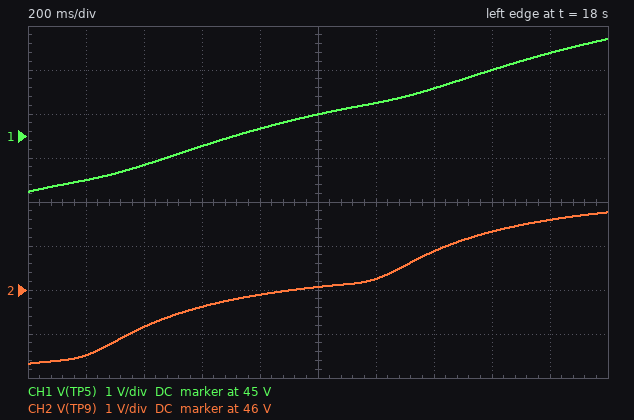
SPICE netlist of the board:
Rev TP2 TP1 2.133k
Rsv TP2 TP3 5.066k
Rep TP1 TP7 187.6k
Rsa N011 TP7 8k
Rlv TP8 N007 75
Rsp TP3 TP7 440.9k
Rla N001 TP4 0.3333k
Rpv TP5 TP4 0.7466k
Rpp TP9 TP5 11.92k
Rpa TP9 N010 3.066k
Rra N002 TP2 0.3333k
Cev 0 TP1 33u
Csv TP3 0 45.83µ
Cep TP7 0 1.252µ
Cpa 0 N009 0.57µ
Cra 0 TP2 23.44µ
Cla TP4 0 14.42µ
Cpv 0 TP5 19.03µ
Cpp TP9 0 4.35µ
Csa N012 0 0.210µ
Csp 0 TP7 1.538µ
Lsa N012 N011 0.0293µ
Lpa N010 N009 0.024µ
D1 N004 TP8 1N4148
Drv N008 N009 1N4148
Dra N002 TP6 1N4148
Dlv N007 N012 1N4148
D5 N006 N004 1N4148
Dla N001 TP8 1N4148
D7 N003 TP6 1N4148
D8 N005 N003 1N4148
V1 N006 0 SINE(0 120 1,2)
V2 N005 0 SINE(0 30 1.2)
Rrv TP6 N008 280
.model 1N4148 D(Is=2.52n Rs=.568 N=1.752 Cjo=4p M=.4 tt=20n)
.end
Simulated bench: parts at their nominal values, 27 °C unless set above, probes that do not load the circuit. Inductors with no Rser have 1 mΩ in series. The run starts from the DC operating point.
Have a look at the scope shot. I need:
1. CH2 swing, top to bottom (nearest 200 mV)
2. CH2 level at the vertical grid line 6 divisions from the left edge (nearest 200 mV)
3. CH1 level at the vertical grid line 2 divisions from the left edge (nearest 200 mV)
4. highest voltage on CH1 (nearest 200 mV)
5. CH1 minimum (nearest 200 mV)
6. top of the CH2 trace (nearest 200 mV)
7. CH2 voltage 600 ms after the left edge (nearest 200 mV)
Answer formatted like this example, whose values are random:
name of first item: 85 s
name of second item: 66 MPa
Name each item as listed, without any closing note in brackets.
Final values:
CH2 swing, top to bottom: 3.4 V
CH2 level at the vertical grid line 6 divisions from the left edge: 46.2 V
CH1 level at the vertical grid line 2 divisions from the left edge: 44.4 V
highest voltage on CH1: 47.2 V
CH1 minimum: 43.8 V
top of the CH2 trace: 47.8 V
CH2 voltage 600 ms after the left edge: 45.6 V
